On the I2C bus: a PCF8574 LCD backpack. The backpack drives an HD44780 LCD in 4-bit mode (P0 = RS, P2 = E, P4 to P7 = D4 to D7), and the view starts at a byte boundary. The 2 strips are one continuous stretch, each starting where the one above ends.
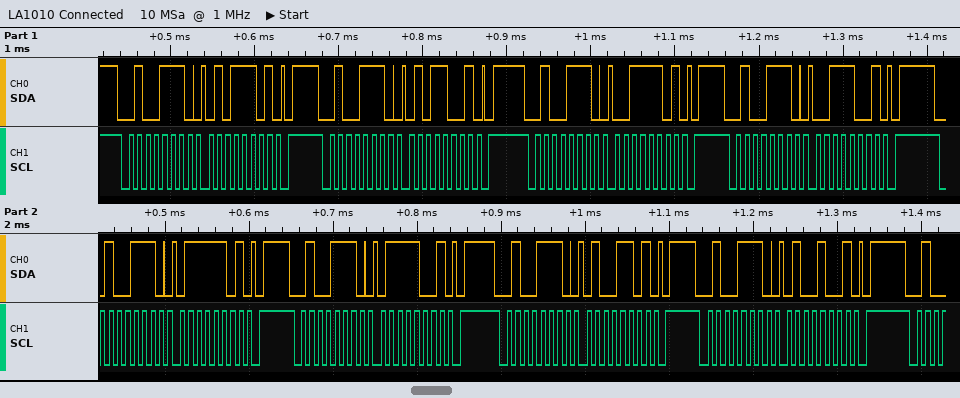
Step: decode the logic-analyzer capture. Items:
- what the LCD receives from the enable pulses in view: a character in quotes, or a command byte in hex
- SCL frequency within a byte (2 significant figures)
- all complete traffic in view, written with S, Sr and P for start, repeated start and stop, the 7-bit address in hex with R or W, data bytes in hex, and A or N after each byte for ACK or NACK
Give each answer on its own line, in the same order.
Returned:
'S' 't'
100 kHz
S 27W A 5D A P S 27W A 59 A P S 27W A 3D A P S 27W A 39 A P S 27W A 7D A P S 27W A 79 A P S 27W A 4D A P S 27W A 49 A P
